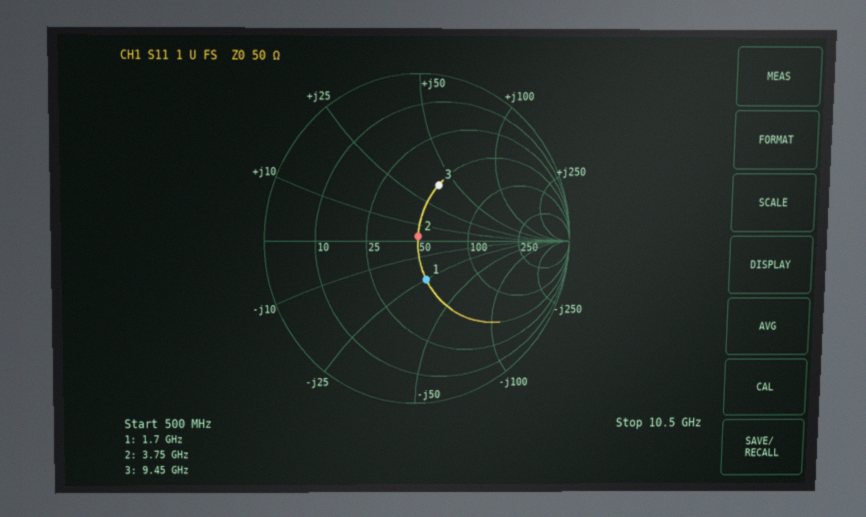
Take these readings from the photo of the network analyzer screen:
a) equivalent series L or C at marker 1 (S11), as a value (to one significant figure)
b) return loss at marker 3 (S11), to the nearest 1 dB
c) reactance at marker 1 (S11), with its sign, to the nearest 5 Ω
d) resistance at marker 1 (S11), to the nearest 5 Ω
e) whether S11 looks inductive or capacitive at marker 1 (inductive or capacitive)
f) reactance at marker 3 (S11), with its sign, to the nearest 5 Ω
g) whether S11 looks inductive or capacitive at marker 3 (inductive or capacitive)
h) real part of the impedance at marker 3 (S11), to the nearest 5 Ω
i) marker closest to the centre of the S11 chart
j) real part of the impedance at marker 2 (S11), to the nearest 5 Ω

4 pF
9 dB
-25 Ω
50 Ω
capacitive
+40 Ω
inductive
50 Ω
marker 2
50 Ω
